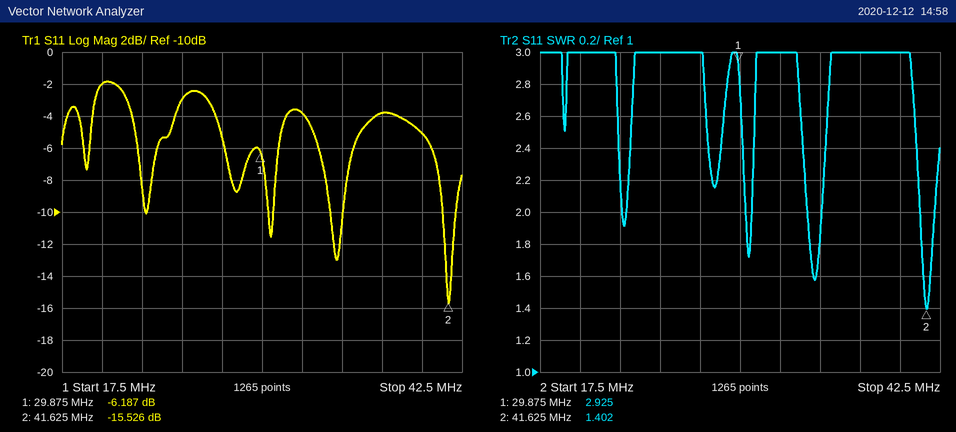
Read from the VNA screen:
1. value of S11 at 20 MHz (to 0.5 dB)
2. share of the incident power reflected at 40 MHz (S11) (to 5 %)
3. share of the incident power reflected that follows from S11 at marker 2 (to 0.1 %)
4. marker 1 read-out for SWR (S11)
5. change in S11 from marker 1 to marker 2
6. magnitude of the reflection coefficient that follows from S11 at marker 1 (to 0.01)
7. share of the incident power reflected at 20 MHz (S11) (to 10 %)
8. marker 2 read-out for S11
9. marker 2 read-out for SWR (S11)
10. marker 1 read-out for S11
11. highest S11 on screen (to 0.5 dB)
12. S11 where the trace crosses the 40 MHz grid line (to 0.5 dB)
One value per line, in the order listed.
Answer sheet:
-2.0 dB
30 %
2.8 %
2.925
-9.339 dB
0.49
60 %
-15.526 dB
1.402
-6.187 dB
-2.0 dB
-5.0 dB
